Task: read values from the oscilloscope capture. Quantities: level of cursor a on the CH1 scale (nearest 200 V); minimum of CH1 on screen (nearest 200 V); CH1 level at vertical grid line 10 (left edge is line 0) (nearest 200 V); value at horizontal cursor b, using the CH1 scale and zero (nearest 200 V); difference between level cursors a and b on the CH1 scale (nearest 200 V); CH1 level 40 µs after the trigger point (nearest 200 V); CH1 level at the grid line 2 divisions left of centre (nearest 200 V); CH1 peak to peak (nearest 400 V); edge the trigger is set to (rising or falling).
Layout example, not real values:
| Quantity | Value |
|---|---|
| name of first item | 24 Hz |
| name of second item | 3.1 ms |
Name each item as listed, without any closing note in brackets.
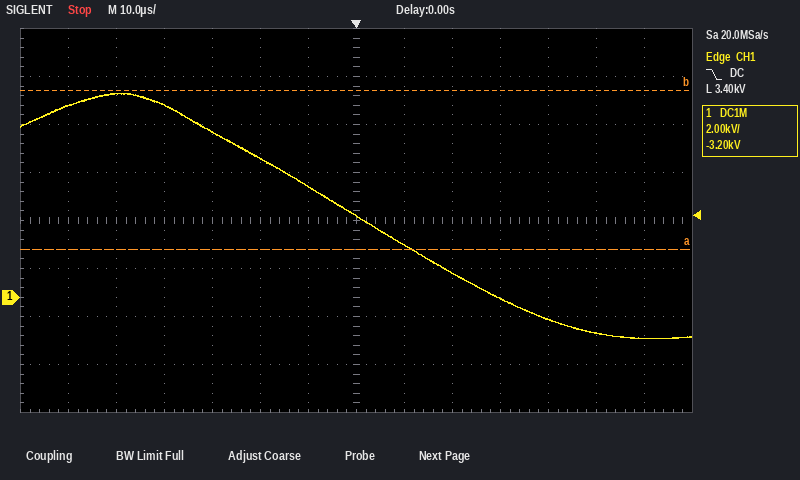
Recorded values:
| Quantity | Value |
|---|---|
| level of cursor a on the CH1 scale | 2.0 kV |
| minimum of CH1 on screen | -1.8 kV |
| CH1 level at vertical grid line 10 (left edge is line 0) | 0.0 kV |
| value at horizontal cursor b, using the CH1 scale and zero | 8.6 kV |
| difference between level cursors a and b on the CH1 scale | 6.6 kV |
| CH1 level 40 µs after the trigger point | -1.0 kV |
| CH1 level at the grid line 2 divisions left of centre | 5.8 kV |
| CH1 peak to peak | 10.4 kV |
| edge the trigger is set to | falling |
